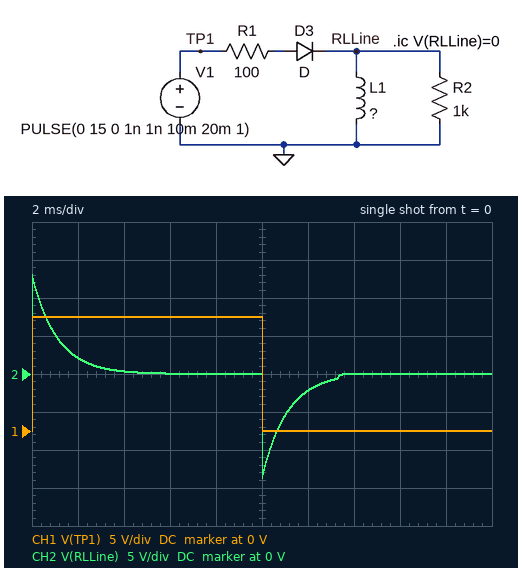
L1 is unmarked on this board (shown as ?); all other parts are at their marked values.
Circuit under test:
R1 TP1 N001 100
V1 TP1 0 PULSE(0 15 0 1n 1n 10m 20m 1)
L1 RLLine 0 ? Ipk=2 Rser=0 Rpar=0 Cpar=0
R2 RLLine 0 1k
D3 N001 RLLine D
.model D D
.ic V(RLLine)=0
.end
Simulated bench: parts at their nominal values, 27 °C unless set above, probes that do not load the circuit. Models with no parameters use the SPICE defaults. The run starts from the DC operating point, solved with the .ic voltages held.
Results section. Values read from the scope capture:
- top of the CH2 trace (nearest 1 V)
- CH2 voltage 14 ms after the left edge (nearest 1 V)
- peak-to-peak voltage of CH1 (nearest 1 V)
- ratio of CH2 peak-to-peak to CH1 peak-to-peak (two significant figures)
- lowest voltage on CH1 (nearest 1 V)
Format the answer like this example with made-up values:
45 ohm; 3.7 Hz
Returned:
13 V; 0 V; 15 V; 1.8; 0 V
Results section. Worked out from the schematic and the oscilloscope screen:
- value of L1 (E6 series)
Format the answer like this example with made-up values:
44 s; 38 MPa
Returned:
100 mH
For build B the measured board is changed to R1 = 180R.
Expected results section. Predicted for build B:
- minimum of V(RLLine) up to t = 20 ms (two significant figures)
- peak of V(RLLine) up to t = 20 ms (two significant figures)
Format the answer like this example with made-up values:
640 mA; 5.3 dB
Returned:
-13 V; 12 V
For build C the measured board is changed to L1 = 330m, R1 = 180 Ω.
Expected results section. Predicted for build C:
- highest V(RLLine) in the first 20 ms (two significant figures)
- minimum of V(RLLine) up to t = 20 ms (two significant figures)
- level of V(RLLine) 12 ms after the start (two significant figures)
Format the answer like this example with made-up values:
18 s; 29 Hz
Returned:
12 V; -13 V; -5.0 V
